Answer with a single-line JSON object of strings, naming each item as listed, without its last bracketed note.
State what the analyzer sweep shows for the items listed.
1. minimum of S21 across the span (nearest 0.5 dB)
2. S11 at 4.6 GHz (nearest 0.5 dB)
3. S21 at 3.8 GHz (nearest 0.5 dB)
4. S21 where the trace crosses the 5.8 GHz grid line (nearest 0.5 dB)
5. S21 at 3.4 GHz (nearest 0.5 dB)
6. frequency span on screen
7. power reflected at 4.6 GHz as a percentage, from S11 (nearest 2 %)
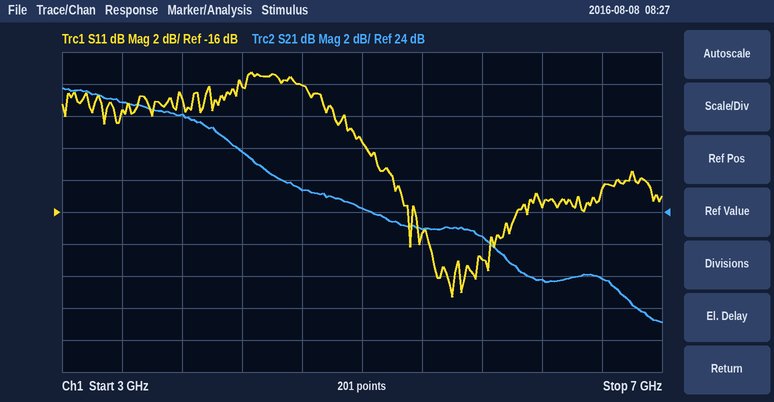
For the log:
{"minimum of S21 across the span": "17.0 dB", "S11 at 4.6 GHz": "-8.0 dB", "S21 at 3.8 GHz": "30.0 dB", "S21 where the trace crosses the 5.8 GHz grid line": "22.5 dB", "S21 at 3.4 GHz": "31.0 dB", "frequency span on screen": "4 GHz", "power reflected at 4.6 GHz as a percentage, from S11": "16 %"}
